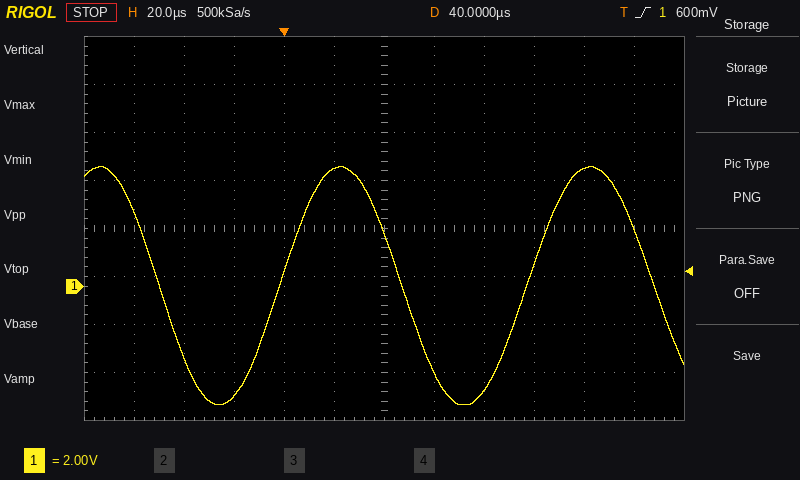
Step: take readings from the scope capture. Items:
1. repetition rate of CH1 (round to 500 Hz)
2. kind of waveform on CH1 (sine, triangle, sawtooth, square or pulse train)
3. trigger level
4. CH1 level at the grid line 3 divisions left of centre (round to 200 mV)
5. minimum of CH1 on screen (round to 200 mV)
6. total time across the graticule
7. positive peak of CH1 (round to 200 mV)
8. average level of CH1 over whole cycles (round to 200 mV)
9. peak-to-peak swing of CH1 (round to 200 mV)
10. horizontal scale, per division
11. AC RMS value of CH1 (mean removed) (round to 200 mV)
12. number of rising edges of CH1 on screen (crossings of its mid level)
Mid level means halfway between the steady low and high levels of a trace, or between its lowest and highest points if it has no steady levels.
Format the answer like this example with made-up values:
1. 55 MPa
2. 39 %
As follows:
1. 10.0 kHz
2. sine
3. 600 mV
4. -4.6 V
5. -5.0 V
6. 240 µs
7. 5.0 V
8. 0.0 V
9. 10.0 V
10. 20 µs
11. 3.6 V
12. 2
